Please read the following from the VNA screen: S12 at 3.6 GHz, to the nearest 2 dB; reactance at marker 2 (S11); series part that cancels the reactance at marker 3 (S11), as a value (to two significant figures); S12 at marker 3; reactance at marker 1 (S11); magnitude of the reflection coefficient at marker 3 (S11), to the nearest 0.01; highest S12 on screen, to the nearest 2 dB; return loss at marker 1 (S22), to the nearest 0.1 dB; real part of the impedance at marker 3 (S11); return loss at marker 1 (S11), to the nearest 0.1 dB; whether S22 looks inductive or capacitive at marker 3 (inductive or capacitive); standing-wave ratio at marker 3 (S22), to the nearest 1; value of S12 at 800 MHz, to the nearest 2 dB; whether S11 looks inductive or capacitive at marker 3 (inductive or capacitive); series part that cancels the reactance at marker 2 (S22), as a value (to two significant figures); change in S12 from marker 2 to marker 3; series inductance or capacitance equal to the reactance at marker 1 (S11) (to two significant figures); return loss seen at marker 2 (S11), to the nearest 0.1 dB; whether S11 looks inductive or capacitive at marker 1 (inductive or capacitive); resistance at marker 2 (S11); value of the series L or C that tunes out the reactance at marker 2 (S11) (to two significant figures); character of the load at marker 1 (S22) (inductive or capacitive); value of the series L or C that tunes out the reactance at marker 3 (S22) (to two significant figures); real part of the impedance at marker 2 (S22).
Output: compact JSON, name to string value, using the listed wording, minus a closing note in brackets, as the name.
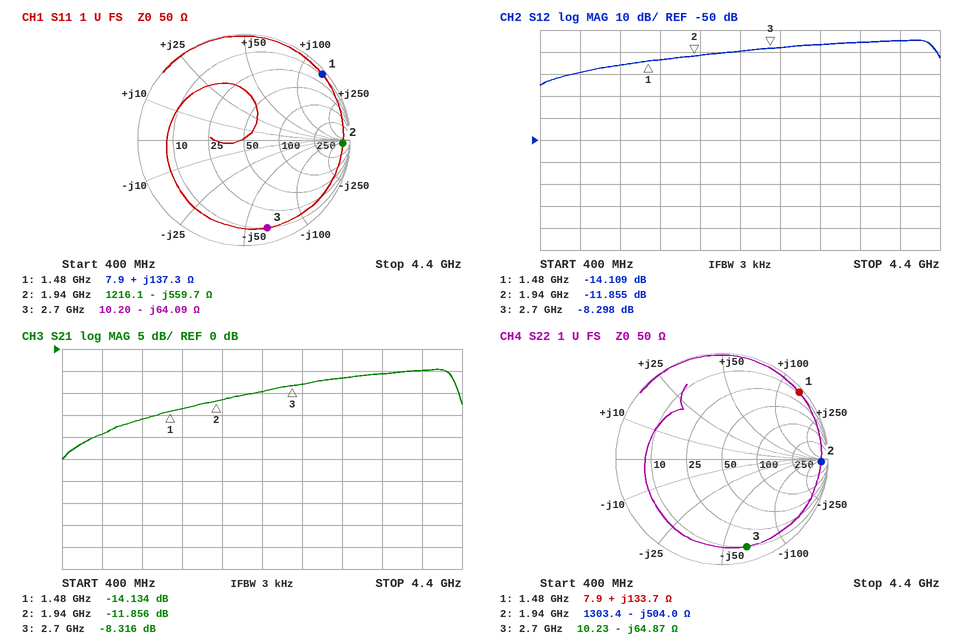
{"S12 at 3.6 GHz, to the nearest 2 dB": "-6 dB", "reactance at marker 2": "-559.7 Ω", "series part that cancels the reactance at marker 3 (S11), as a value": "3.8 nH", "S12 at marker 3": "-8.298 dB", "reactance at marker 1": "+137.3 Ω", "magnitude of the reflection coefficient at marker 3 (S11), to the nearest 0.01": "0.86", "highest S12 on screen, to the nearest 2 dB": "-4 dB", "return loss at marker 1 (S22), to the nearest 0.1 dB": "0.3 dB", "real part of the impedance at marker 3": "10.20 Ω", "return loss at marker 1 (S11), to the nearest 0.1 dB": "0.3 dB", "whether S22 looks inductive or capacitive at marker 3": "capacitive", "standing-wave ratio at marker 3 (S22), to the nearest 1": "13", "value of S12 at 800 MHz, to the nearest 2 dB": "-20 dB", "whether S11 looks inductive or capacitive at marker 3": "capacitive", "series part that cancels the reactance at marker 2 (S22), as a value": "41 nH", "change in S12 from marker 2 to marker 3": "3.557 dB", "series inductance or capacitance equal to the reactance at marker 1 (S11)": "15 nH", "return loss seen at marker 2 (S11), to the nearest 0.1 dB": "0.6 dB", "whether S11 looks inductive or capacitive at marker 1": "inductive", "resistance at marker 2": "1216.1 Ω", "value of the series L or C that tunes out the reactance at marker 2 (S11)": "46 nH", "character of the load at marker 1 (S22)": "inductive", "value of the series L or C that tunes out the reactance at marker 3 (S22)": "3.8 nH", "real part of the impedance at marker 2": "1303.4 Ω"}
